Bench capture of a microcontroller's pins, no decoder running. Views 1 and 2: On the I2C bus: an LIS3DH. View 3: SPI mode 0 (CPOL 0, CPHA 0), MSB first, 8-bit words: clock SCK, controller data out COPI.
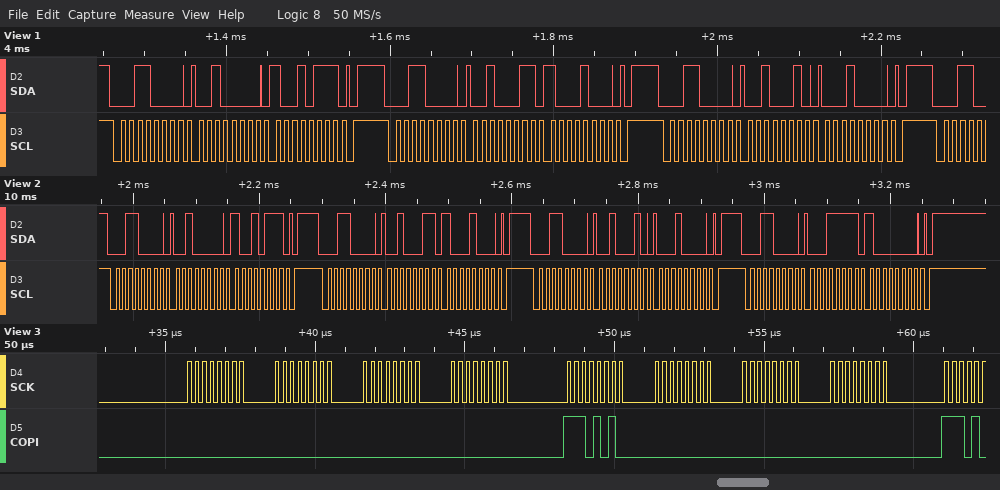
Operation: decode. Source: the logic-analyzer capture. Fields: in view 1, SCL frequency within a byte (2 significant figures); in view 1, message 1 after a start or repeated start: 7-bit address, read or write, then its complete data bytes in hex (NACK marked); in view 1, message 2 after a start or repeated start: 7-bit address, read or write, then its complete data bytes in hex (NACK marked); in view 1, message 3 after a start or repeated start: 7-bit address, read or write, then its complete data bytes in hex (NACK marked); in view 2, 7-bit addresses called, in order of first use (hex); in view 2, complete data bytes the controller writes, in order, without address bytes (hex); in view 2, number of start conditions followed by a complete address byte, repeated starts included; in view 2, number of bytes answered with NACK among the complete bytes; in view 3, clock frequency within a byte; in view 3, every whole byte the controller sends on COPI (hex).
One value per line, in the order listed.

100 kHz
0x18 write: 20 97
0x18 write: 23 88
0x18 write: 22 10
0x18
20 97 23 88 22 10 1F 80
4
0
4 MHz
0x00 0x00 0x00 0x00 0xEA 0x00 0x00 0x00
